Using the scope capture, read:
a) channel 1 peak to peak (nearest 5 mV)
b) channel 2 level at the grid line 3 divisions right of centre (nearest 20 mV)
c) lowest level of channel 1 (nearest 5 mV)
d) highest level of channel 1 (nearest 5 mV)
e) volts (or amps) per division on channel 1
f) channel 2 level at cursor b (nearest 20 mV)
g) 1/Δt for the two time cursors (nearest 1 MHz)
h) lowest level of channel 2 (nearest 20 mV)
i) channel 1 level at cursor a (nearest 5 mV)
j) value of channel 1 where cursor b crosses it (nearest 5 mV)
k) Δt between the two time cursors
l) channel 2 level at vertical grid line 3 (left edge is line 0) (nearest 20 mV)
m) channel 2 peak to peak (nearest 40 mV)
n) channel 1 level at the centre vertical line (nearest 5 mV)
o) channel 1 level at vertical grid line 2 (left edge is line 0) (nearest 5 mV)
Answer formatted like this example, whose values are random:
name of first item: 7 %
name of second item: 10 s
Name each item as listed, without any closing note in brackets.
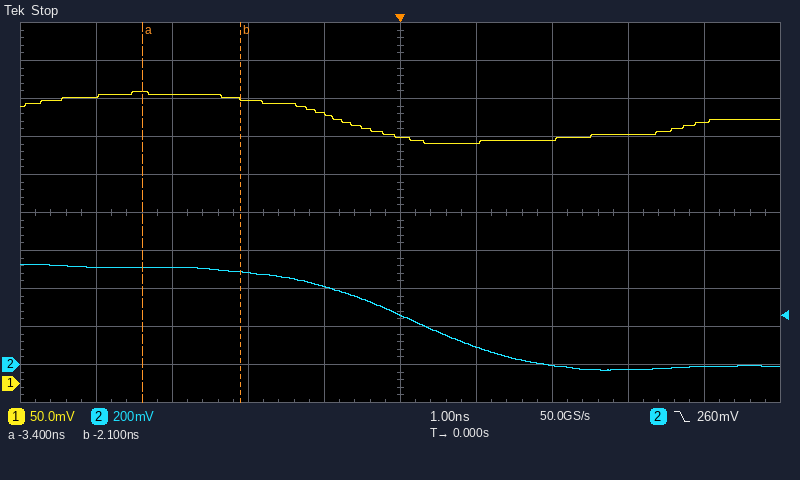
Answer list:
channel 1 peak to peak: 70 mV
channel 2 level at the grid line 3 divisions right of centre: -20 mV
lowest level of channel 1: 315 mV
highest level of channel 1: 385 mV
volts (or amps) per division on channel 1: 50 mV
channel 2 level at cursor b: 480 mV
1/Δt for the two time cursors: 769 MHz
lowest level of channel 2: -40 mV
channel 1 level at cursor a: 385 mV
value of channel 1 where cursor b crosses it: 375 mV
Δt between the two time cursors: 1.3 ns
channel 2 level at vertical grid line 3 (left edge is line 0): 480 mV
channel 2 peak to peak: 560 mV
channel 1 level at the centre vertical line: 325 mV
channel 1 level at vertical grid line 2 (left edge is line 0): 380 mV
